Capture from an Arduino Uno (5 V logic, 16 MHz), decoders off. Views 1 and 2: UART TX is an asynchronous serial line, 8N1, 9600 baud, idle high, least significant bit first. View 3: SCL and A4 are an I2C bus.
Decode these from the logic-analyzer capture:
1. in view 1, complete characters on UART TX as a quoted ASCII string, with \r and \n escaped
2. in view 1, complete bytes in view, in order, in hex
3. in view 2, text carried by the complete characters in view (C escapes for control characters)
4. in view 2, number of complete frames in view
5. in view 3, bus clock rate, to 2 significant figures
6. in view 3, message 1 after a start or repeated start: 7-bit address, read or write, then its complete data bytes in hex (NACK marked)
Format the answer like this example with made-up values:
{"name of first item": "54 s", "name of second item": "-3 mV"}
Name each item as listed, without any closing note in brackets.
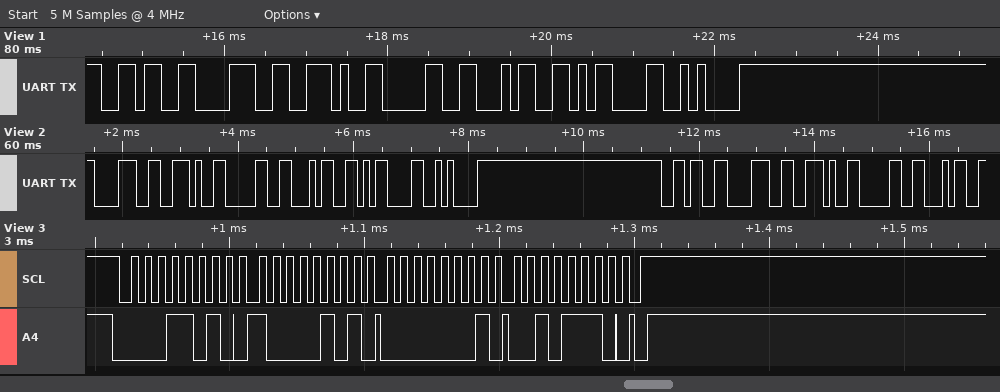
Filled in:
{"in view 1, complete characters on UART TX as a quoted ASCII string, with \\r and \\n escaped": "\"68.04\\r\\n\"", "in view 1, complete bytes in view, in order, in hex": "36 38 2E 30 34 0D 0A", "in view 2, text carried by the complete characters in view": "\"8.04\\r\\n68.04\"", "in view 2, number of complete frames in view": "11", "in view 3, bus clock rate, to 2 significant figures": "100 kHz", "in view 3, message 1 after a start or repeated start: 7-bit address, read or write, then its complete data bytes in hex": "0x0D write: 85 01 2E"}
